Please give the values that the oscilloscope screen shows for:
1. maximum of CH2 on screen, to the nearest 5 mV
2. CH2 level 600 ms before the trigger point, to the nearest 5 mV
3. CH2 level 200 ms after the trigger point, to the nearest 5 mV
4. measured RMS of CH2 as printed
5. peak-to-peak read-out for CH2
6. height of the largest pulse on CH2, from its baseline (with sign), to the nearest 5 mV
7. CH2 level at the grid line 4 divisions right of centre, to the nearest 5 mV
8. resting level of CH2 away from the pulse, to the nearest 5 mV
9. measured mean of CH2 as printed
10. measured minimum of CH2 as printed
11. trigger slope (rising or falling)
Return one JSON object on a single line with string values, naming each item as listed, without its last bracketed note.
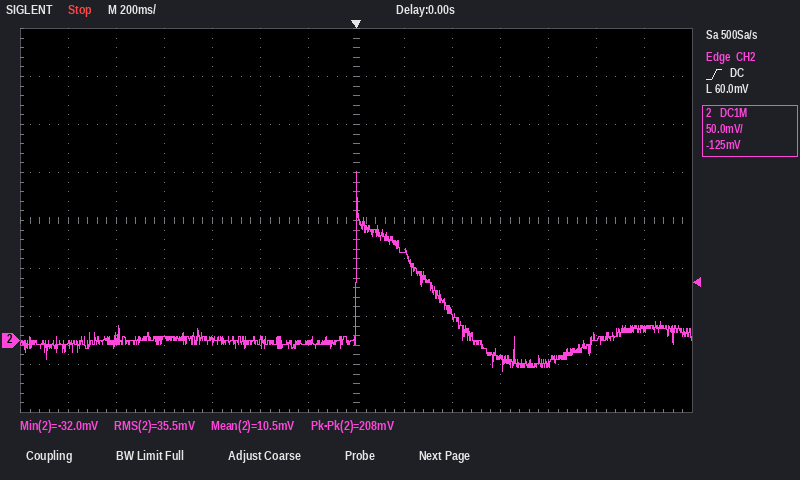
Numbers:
{"maximum of CH2 on screen, to the nearest 5 mV": "175 mV", "CH2 level 600 ms before the trigger point, to the nearest 5 mV": "0 mV", "CH2 level 200 ms after the trigger point, to the nearest 5 mV": "95 mV", "measured RMS of CH2 as printed": "35.5 mV", "peak-to-peak read-out for CH2": "208 mV", "height of the largest pulse on CH2, from its baseline (with sign), to the nearest 5 mV": "+175 mV", "CH2 level at the grid line 4 divisions right of centre, to the nearest 5 mV": "-25 mV", "resting level of CH2 away from the pulse, to the nearest 5 mV": "0 mV", "measured mean of CH2 as printed": "10.5 mV", "measured minimum of CH2 as printed": "-32.0 mV", "trigger slope": "rising"}
